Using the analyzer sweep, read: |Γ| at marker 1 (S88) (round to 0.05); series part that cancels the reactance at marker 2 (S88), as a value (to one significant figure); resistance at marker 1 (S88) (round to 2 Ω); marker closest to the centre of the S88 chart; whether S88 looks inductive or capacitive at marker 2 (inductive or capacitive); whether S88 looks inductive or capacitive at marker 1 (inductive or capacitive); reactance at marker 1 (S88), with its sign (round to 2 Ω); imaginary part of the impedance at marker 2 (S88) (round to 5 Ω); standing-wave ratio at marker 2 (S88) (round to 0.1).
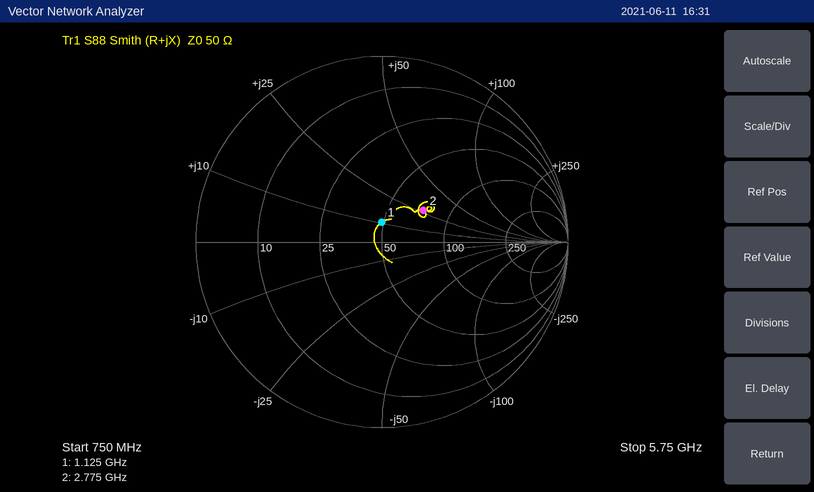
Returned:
0.10
2 pF
48 Ω
marker 1
inductive
inductive
+10 Ω
+25 Ω
1.8
